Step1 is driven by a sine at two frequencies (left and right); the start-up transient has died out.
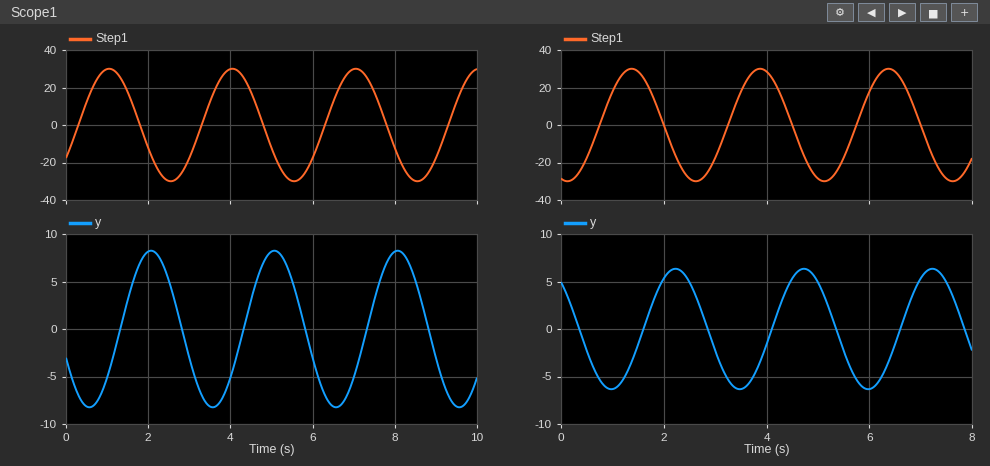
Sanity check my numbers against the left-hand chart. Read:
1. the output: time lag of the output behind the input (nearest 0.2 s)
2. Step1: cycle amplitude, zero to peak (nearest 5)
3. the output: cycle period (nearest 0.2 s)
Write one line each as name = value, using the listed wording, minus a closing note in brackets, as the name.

the output: time lag of the output behind the input = 1.0 s
Step1: cycle amplitude, zero to peak = 30
the output: cycle period = 3.0 s
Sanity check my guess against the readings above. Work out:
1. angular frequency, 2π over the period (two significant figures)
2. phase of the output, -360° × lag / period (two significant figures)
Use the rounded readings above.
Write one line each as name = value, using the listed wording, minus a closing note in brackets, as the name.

angular frequency, 2π over the period = 2.1 rad/s
phase of the output, -360° × lag / period = -120°
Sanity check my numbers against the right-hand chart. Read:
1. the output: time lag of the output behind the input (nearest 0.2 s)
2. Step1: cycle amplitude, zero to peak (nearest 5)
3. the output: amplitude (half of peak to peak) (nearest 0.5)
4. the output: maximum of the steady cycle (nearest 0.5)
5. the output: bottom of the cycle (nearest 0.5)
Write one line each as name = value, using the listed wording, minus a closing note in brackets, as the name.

the output: time lag of the output behind the input = 0.8 s
Step1: cycle amplitude, zero to peak = 30
the output: amplitude (half of peak to peak) = 6.5
the output: maximum of the steady cycle = 6.5
the output: bottom of the cycle = -6.5
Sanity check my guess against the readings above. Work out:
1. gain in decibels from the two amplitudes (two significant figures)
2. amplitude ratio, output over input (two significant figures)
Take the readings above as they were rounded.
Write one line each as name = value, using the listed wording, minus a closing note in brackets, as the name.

gain in decibels from the two amplitudes = -13 dB
amplitude ratio, output over input = 0.22
